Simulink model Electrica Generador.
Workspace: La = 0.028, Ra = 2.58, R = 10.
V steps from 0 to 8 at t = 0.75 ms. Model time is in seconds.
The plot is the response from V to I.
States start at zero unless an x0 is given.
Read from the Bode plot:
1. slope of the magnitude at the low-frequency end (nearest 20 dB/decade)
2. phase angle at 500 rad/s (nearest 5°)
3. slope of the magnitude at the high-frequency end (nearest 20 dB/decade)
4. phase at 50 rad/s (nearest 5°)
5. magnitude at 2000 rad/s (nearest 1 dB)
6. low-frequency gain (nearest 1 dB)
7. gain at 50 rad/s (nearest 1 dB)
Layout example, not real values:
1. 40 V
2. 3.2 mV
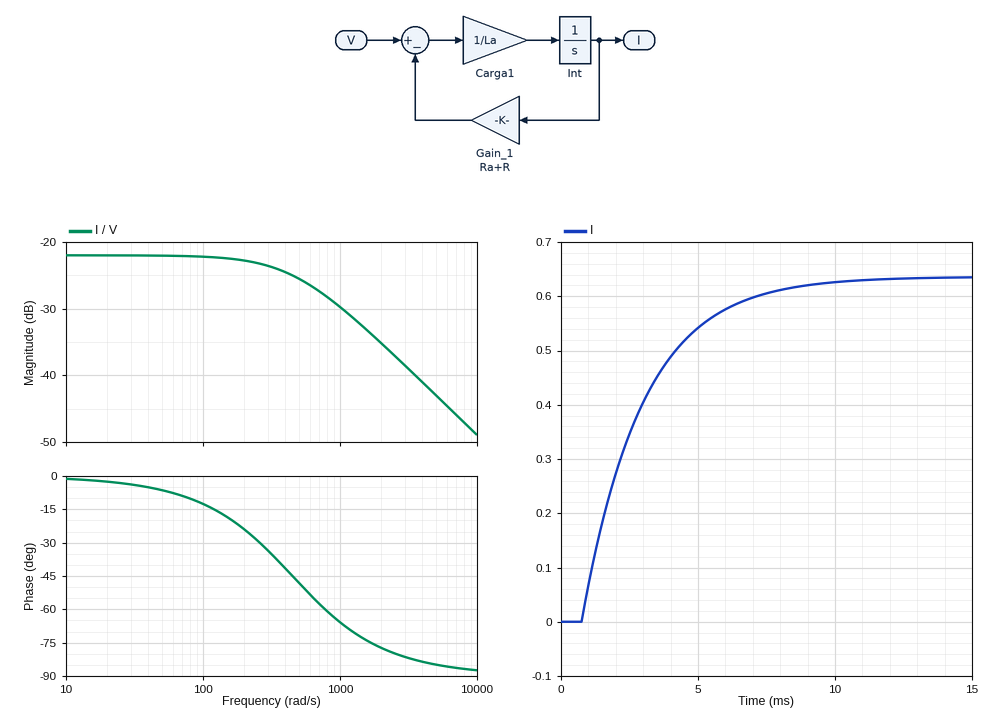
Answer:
1. 0 dB/decade
2. -50°
3. -20 dB/decade
4. -5°
5. -35 dB
6. -22 dB
7. -22 dB
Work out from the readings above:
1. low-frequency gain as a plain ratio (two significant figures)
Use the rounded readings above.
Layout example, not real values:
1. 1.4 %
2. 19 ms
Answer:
1. 0.079
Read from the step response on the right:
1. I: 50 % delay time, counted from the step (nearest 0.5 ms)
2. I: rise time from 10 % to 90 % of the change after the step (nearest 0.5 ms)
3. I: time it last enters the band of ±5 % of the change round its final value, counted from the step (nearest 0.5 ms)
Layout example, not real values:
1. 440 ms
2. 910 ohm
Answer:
1. 1.5 ms
2. 5.0 ms
3. 6.5 ms
